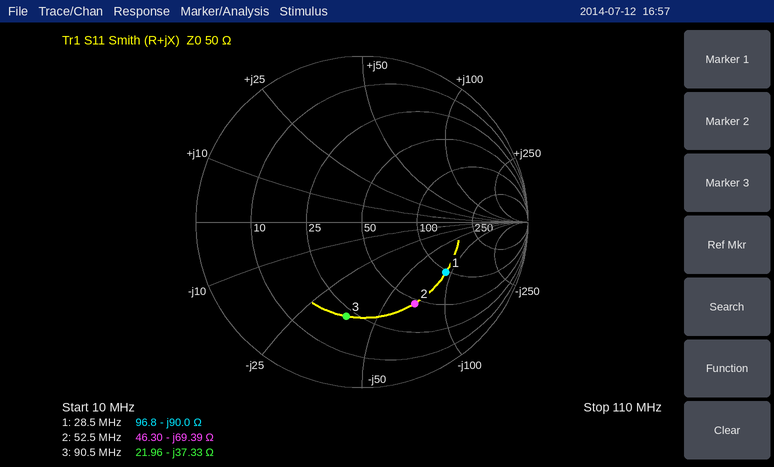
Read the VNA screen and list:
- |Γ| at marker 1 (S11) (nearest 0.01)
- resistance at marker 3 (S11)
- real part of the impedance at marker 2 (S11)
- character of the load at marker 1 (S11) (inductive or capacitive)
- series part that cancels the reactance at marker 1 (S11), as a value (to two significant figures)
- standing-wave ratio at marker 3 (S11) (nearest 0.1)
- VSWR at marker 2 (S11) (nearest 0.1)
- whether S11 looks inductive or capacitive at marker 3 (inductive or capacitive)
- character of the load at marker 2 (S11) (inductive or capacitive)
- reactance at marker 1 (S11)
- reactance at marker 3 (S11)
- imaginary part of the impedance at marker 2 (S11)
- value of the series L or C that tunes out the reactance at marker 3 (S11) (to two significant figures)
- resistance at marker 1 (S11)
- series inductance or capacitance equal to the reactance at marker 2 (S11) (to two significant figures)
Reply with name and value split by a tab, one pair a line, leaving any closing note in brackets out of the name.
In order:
|Γ| at marker 1 (S11)	0.59
resistance at marker 3	21.96 Ω
real part of the impedance at marker 2	46.30 Ω
character of the load at marker 1 (S11)	capacitive
series part that cancels the reactance at marker 1 (S11), as a value	500 nH
standing-wave ratio at marker 3 (S11)	3.7
VSWR at marker 2 (S11)	3.8
whether S11 looks inductive or capacitive at marker 3	capacitive
character of the load at marker 2 (S11)	capacitive
reactance at marker 1	-90.0 Ω
reactance at marker 3	-37.33 Ω
imaginary part of the impedance at marker 2	-69.39 Ω
value of the series L or C that tunes out the reactance at marker 3 (S11)	66 nH
resistance at marker 1	96.8 Ω
series inductance or capacitance equal to the reactance at marker 2 (S11)	44 pF
